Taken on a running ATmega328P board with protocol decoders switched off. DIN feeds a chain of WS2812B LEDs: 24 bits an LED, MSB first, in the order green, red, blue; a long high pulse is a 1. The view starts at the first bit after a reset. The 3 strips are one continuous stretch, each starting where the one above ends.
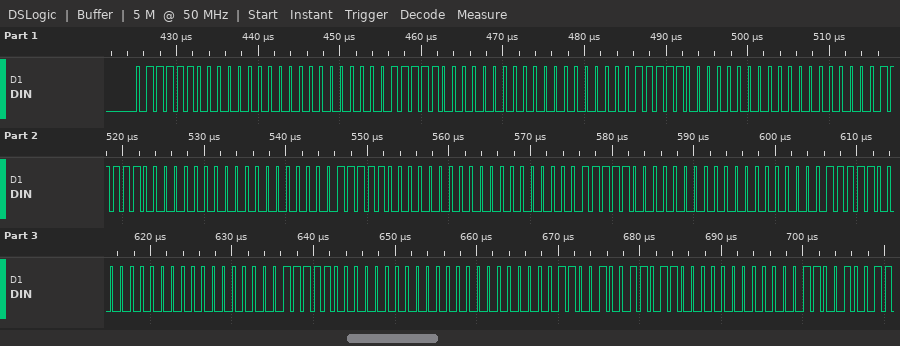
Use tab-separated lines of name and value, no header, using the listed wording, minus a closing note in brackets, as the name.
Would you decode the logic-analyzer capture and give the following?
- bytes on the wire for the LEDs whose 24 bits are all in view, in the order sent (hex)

bytes on the wire for the LEDs whose 24 bits are all in view, in the order sent	7C 00 00 7C 00 00 7C 00 00 7C 00 00 7C 00 00 7C 00 00 7C 00 00 7C 00 00 0C 9B 00
